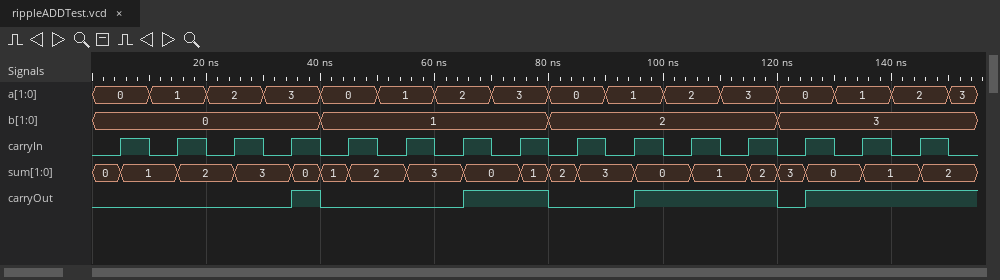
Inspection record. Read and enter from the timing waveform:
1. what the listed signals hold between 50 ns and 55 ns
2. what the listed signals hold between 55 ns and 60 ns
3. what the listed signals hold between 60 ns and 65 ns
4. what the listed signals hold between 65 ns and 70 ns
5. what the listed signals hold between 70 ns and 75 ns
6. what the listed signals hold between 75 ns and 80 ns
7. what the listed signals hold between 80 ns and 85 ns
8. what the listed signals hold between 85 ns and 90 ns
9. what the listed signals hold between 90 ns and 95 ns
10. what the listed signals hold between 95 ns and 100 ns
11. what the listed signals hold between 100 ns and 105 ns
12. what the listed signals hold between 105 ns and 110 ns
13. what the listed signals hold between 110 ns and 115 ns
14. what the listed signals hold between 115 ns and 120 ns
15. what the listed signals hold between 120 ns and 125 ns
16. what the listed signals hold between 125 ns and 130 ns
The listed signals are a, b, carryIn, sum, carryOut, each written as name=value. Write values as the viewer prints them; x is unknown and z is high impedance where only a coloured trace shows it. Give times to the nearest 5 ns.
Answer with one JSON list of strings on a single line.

["a=1, b=1, carryIn=0, sum=2, carryOut=0", "a=1, b=1, carryIn=1, sum=3, carryOut=0", "a=2, b=1, carryIn=0, sum=3, carryOut=0", "a=2, b=1, carryIn=1, sum=0, carryOut=1", "a=3, b=1, carryIn=0, sum=0, carryOut=1", "a=3, b=1, carryIn=1, sum=1, carryOut=1", "a=0, b=2, carryIn=0, sum=2, carryOut=0", "a=0, b=2, carryIn=1, sum=3, carryOut=0", "a=1, b=2, carryIn=0, sum=3, carryOut=0", "a=1, b=2, carryIn=1, sum=0, carryOut=1", "a=2, b=2, carryIn=0, sum=0, carryOut=1", "a=2, b=2, carryIn=1, sum=1, carryOut=1", "a=3, b=2, carryIn=0, sum=1, carryOut=1", "a=3, b=2, carryIn=1, sum=2, carryOut=1", "a=0, b=3, carryIn=0, sum=3, carryOut=0", "a=0, b=3, carryIn=1, sum=0, carryOut=1"]
